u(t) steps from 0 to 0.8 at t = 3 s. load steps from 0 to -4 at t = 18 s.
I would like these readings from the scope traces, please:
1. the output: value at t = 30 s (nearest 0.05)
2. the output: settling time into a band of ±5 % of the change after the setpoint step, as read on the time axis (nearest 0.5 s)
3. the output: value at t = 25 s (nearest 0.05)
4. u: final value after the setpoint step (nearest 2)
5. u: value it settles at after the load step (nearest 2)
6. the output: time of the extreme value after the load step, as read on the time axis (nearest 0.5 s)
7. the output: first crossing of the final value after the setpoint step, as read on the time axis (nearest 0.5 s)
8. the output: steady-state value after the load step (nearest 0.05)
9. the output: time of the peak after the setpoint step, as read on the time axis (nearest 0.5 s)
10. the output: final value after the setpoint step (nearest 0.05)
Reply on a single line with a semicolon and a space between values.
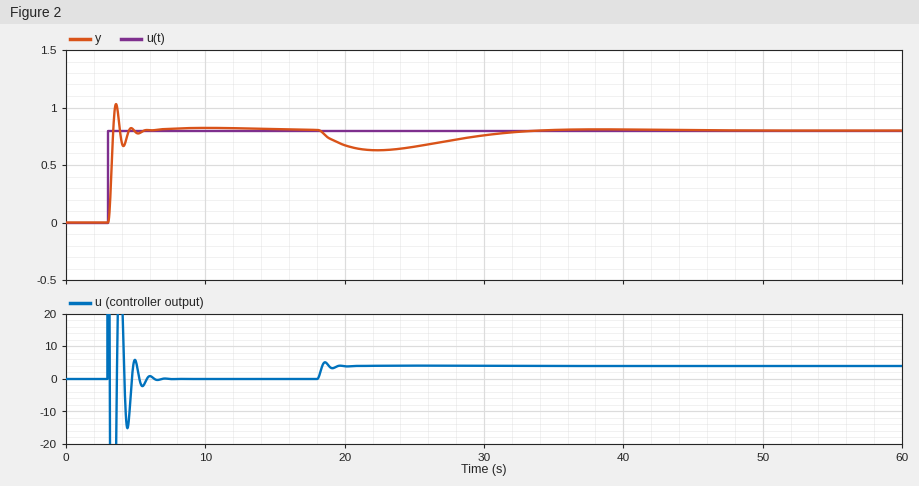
0.75; 4.5 s; 0.65; 0; 4; 22.5 s; 3.5 s; 0.80; 3.5 s; 0.80
